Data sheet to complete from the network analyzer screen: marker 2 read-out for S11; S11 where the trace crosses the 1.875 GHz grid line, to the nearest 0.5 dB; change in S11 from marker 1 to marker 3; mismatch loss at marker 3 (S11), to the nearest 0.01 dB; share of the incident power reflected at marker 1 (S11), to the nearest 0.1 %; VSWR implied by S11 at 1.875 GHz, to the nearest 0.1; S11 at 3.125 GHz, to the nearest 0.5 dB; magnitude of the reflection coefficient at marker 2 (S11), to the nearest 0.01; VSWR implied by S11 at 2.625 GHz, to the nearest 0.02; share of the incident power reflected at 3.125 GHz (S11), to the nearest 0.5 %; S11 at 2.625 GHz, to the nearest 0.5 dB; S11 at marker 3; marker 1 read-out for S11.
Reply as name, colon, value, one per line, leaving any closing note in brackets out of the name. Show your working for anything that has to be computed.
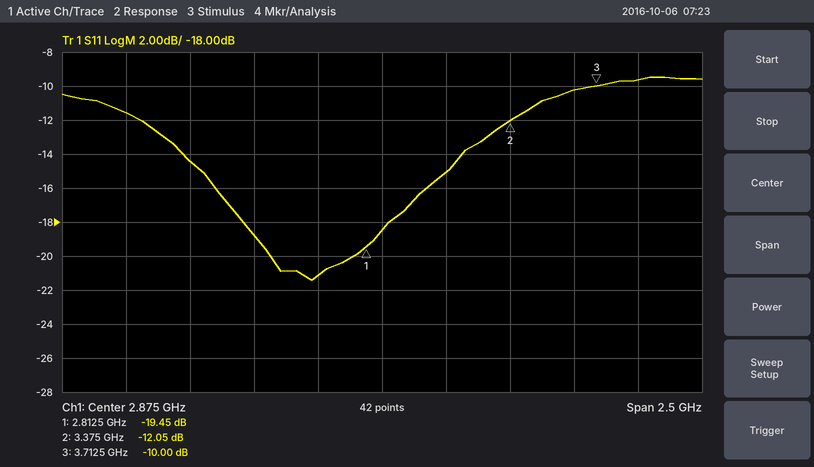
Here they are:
marker 2 read-out for S11: -12.05 dB
S11 where the trace crosses the 1.875 GHz grid line, to the nearest 0.5 dB: -11.5 dB
change in S11 from marker 1 to marker 3: -10 − (-19.45) = 9.45 dB
mismatch loss at marker 3 (S11), to the nearest 0.01 dB: −10 log10(1 − 10^(-10/10)) ≈ 0.46 dB
share of the incident power reflected at marker 1 (S11), to the nearest 0.1 %: 10^(-19.45/10) ≈ 1.1 %
VSWR implied by S11 at 1.875 GHz, to the nearest 0.1: |Γ| = 10^(-11.5/20) = 0.2661; VSWR = (1 + 0.2661)/(1 − 0.2661) ≈ 1.7
S11 at 3.125 GHz, to the nearest 0.5 dB: -15.0 dB
magnitude of the reflection coefficient at marker 2 (S11), to the nearest 0.01: 10^(-12.05/20) ≈ 0.25
VSWR implied by S11 at 2.625 GHz, to the nearest 0.02: |Γ| = 10^(-21/20) = 0.0891; VSWR = (1 + 0.0891)/(1 − 0.0891) ≈ 1.20
share of the incident power reflected at 3.125 GHz (S11), to the nearest 0.5 %: 10^(-15/10) ≈ 3.16 %, so 3.0 % to the nearest 0.5 %
S11 at 2.625 GHz, to the nearest 0.5 dB: -21.0 dB
S11 at marker 3: -10.00 dB
marker 1 read-out for S11: -19.45 dB
